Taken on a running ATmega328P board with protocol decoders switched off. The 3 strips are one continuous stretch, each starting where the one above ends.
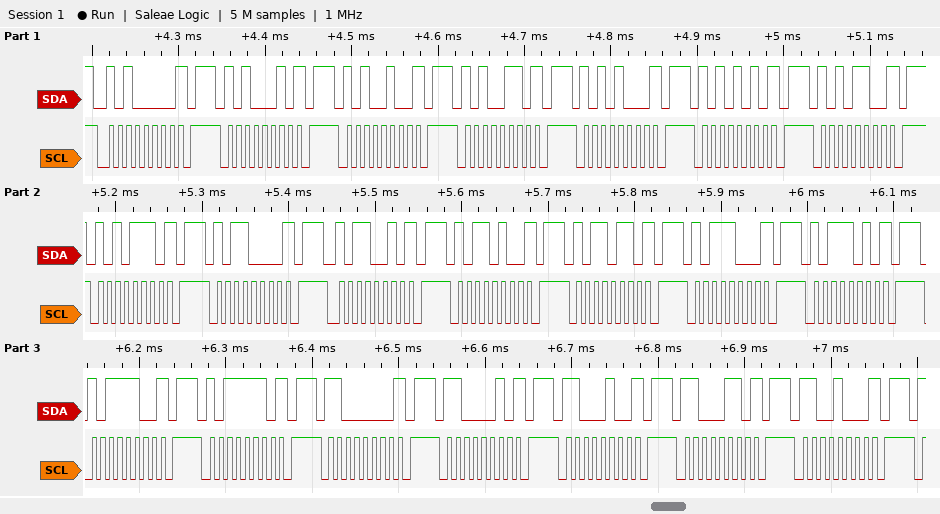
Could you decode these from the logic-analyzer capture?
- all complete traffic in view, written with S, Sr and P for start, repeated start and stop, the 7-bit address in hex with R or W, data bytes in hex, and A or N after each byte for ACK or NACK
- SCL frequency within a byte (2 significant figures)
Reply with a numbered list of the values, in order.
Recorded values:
1. S 50W N P S 51W N P S 52W N P S 53W N P S 54W N P S 55W N P S 56W N P S 57W N P S 58W N P S 59W N P S 5AW N P S 5BW N P S 5CW N P S 5DW N P S 5EW N P S 5FW N P S 60W N P S 61W N P S 62W N P S 63W N P S 64W N P
2. 100 kHz
